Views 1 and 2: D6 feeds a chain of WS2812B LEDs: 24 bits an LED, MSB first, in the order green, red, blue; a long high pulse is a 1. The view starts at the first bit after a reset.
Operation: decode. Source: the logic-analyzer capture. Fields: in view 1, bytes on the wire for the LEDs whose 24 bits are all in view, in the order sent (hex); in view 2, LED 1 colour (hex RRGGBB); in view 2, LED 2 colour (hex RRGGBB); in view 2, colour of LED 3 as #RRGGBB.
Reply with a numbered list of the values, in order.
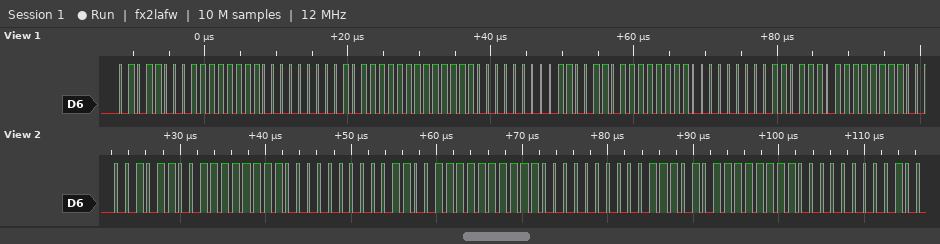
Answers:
1. 58 FF 00 5F FF 00 66 FF 00
2. #FF2C00
3. #FF3300
4. #FF3A00
